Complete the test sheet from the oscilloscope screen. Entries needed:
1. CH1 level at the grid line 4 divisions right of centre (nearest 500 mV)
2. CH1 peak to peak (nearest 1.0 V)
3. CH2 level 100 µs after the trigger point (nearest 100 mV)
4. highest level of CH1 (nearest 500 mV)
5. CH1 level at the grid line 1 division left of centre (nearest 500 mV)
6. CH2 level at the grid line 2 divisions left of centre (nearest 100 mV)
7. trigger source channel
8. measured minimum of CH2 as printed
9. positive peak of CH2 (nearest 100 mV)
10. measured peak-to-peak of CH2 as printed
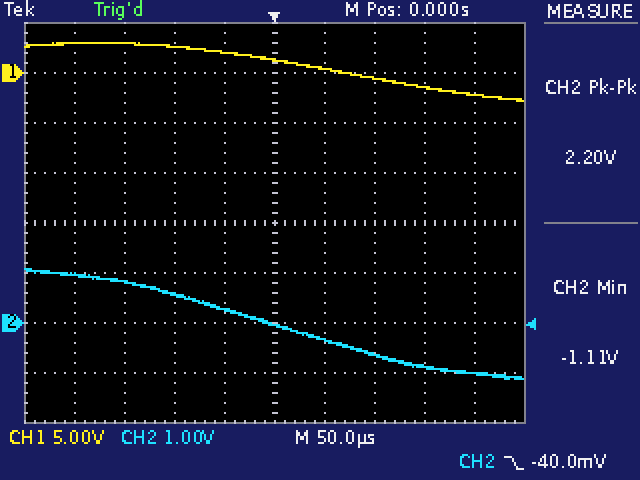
-2.0 V
6.0 V
-600 mV
3.0 V
2.0 V
600 mV
CH2
-1.11 V
1.1 V
2.20 V
